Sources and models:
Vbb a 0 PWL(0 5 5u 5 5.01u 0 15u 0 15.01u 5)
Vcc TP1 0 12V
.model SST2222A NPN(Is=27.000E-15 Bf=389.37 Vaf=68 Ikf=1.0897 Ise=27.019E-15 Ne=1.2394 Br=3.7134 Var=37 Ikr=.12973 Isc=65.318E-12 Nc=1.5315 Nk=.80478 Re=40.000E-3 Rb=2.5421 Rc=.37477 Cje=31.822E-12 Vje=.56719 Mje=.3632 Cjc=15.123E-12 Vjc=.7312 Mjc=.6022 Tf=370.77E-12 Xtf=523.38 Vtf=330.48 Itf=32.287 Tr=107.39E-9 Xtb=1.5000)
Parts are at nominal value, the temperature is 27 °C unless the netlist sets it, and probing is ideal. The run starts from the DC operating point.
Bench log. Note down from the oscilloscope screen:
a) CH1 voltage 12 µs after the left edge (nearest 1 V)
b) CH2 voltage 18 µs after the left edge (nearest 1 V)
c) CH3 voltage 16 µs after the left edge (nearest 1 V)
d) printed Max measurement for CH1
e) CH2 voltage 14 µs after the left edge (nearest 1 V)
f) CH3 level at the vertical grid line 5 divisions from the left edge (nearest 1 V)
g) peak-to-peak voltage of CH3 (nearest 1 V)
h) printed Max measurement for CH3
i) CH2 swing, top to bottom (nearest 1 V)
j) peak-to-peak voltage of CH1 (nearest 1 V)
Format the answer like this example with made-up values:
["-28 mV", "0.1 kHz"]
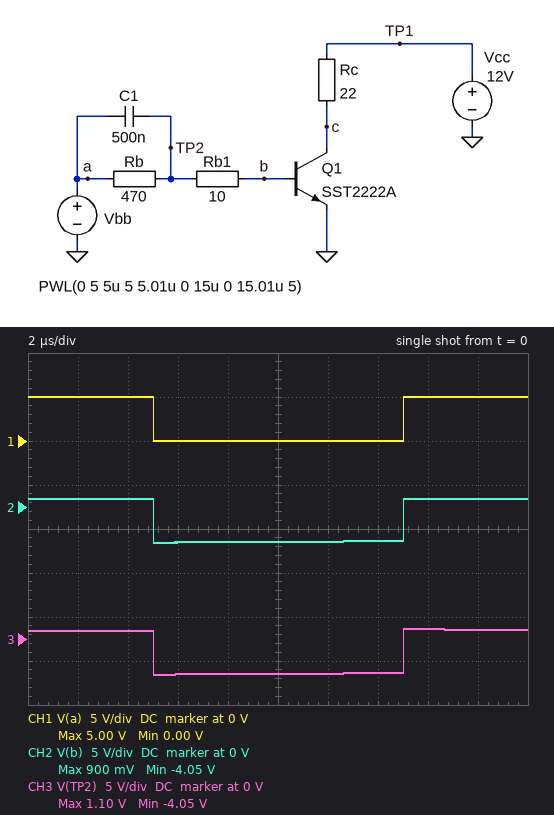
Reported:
["0 V", "1 V", "1 V", "5.00 V", "-4 V", "-4 V", "5 V", "1.10 V", "5 V", "5 V"]
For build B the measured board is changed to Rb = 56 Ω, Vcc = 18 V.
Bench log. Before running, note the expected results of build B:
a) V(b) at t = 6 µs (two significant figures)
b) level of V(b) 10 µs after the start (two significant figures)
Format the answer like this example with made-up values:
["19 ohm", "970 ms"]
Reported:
["-3.2 V", "-2.8 V"]
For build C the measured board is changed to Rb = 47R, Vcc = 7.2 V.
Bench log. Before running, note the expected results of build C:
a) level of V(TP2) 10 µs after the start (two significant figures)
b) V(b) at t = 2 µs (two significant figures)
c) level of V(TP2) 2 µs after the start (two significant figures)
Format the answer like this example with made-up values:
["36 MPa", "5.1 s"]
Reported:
["-2.6 V", "1.0 V", "1.7 V"]
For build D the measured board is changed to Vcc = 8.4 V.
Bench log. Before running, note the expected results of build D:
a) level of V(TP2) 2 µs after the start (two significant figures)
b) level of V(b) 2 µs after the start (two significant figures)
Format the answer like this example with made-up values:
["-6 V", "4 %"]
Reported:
["930 mV", "840 mV"]
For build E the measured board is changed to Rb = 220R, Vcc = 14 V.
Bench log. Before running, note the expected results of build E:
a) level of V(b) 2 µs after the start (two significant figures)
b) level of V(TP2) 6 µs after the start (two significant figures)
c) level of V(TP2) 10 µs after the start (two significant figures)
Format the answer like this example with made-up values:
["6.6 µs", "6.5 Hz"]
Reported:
["900 mV", "-3.9 V", "-3.7 V"]
